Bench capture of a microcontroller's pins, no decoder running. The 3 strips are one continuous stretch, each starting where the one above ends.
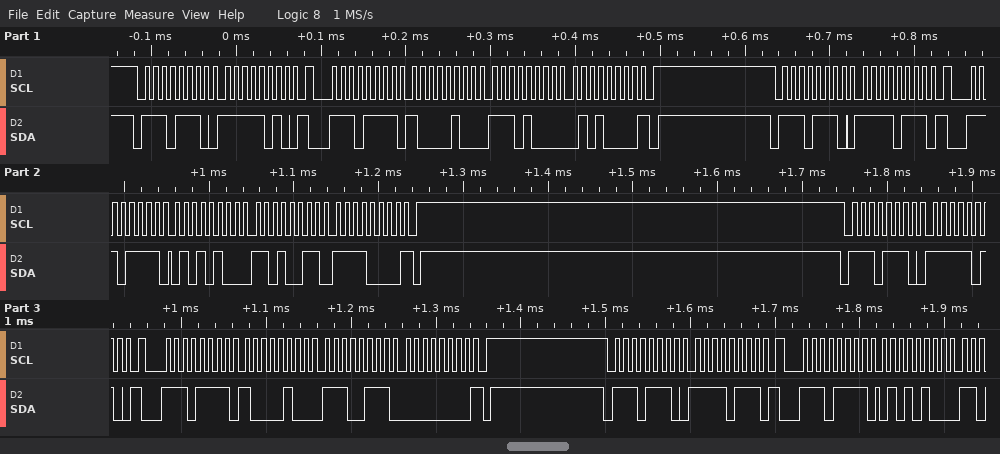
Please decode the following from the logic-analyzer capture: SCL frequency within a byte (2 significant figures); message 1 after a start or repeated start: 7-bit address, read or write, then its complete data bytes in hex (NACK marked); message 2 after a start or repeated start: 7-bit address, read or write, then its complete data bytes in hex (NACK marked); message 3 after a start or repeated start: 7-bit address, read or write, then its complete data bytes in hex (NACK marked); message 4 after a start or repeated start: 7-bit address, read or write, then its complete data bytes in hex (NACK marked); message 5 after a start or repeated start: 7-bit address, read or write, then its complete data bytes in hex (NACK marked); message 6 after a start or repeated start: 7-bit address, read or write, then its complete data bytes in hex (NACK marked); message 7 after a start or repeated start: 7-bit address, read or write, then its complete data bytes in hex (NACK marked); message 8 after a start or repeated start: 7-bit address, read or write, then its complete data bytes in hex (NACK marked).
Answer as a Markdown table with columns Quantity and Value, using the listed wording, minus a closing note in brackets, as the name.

| Quantity | Value |
|---|---|
| SCL frequency within a byte | 100 kHz |
| message 1 after a start or repeated start: 7-bit address, read or write, then its complete data bytes in hex | 0x77 write: FA |
| message 2 after a start or repeated start: 7-bit address, read or write, then its complete data bytes in hex | 0x77 read: 84 E8 50 NACK |
| message 3 after a start or repeated start: 7-bit address, read or write, then its complete data bytes in hex | 0x77 write: F7 |
| message 4 after a start or repeated start: 7-bit address, read or write, then its complete data bytes in hex | 0x77 read: 54 D3 F0 NACK |
| message 5 after a start or repeated start: 7-bit address, read or write, then its complete data bytes in hex | 0x77 write: FA |
| message 6 after a start or repeated start: 7-bit address, read or write, then its complete data bytes in hex | 0x77 read: 84 E7 00 NACK |
| message 7 after a start or repeated start: 7-bit address, read or write, then its complete data bytes in hex | 0x77 write: F7 |
| message 8 after a start or repeated start: 7-bit address, read or write, then its complete data bytes in hex | 0x77 read: 54 |
